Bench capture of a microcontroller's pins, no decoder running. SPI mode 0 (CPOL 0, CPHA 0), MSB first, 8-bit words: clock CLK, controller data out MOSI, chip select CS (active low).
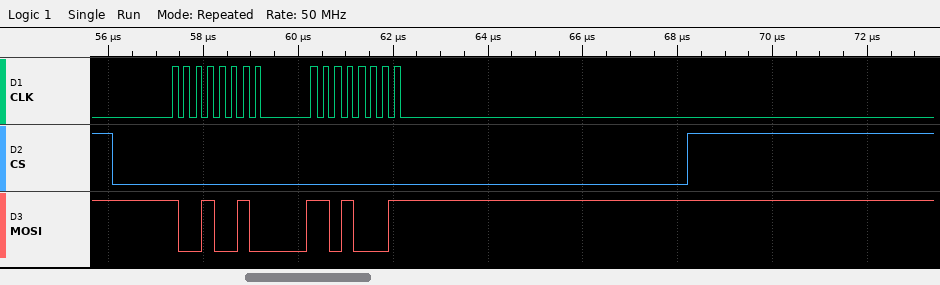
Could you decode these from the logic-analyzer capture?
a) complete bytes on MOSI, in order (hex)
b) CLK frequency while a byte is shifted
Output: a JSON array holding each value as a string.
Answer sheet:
["92 D1", "4 MHz"]
